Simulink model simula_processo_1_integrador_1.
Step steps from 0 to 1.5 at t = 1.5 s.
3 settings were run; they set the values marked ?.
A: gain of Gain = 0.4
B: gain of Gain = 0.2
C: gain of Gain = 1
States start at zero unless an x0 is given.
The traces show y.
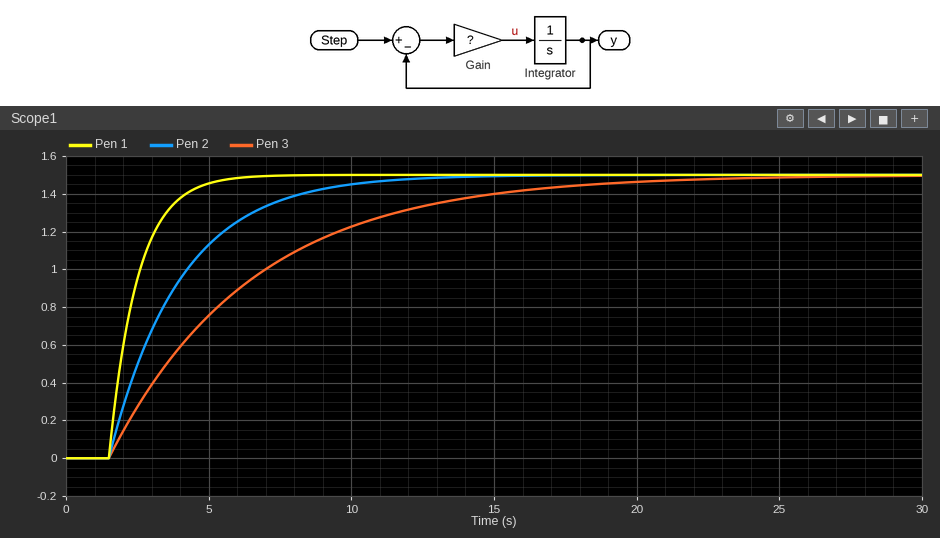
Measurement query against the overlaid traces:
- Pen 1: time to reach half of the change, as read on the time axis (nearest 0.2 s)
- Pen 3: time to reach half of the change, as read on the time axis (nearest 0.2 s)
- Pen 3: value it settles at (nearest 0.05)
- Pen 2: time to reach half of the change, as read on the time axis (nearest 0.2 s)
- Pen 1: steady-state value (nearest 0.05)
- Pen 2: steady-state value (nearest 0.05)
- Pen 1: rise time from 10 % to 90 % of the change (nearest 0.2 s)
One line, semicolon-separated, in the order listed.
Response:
2.2 s; 5.0 s; 1.50; 3.2 s; 1.50; 1.50; 2.2 s
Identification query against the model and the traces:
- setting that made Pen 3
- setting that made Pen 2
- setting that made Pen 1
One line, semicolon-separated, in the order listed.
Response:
B; A; C
